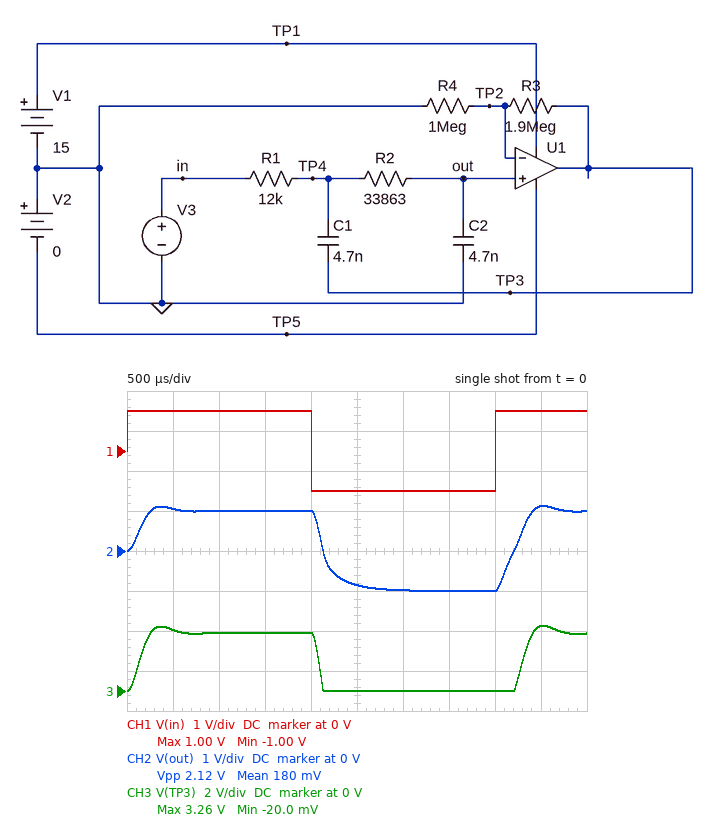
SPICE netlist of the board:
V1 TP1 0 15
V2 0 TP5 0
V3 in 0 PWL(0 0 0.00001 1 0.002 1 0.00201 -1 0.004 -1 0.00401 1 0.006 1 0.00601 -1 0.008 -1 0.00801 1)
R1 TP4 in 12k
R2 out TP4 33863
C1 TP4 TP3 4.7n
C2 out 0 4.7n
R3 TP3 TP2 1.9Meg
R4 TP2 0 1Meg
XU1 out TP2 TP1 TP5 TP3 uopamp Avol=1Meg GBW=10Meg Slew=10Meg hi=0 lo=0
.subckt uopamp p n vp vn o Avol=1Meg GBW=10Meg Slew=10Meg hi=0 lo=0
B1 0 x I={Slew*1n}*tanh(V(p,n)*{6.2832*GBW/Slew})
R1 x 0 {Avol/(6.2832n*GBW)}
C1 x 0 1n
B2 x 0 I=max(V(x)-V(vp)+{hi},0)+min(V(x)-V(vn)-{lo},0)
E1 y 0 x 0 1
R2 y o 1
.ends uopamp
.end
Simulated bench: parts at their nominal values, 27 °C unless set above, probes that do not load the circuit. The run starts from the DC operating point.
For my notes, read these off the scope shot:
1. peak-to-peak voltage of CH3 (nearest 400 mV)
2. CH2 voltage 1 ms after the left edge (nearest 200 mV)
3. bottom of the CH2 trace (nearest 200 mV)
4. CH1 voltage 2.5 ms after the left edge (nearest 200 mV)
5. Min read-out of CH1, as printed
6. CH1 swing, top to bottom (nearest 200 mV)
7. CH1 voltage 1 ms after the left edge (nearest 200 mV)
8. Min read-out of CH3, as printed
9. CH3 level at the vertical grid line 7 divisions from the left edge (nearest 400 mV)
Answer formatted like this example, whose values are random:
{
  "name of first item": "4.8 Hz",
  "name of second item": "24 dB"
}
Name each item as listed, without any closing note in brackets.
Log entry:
{
  "peak-to-peak voltage of CH3": "3.2 V",
  "CH2 voltage 1 ms after the left edge": "1.0 V",
  "bottom of the CH2 trace": "-1.0 V",
  "CH1 voltage 2.5 ms after the left edge": "-1.0 V",
  "Min read-out of CH1, as printed": "-1.00 V",
  "CH1 swing, top to bottom": "2.0 V",
  "CH1 voltage 1 ms after the left edge": "1.0 V",
  "Min read-out of CH3, as printed": "-20.0 mV",
  "CH3 level at the vertical grid line 7 divisions from the left edge": "0 V"
}
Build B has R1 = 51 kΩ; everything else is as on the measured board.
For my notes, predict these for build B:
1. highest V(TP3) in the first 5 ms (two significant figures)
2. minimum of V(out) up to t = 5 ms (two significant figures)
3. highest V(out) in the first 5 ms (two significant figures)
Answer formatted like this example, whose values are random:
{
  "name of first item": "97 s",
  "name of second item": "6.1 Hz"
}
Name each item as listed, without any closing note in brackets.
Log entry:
{
  "highest V(TP3) in the first 5 ms": "7.7 V",
  "minimum of V(out) up to t = 5 ms": "-1.2 V",
  "highest V(out) in the first 5 ms": "2.7 V"
}
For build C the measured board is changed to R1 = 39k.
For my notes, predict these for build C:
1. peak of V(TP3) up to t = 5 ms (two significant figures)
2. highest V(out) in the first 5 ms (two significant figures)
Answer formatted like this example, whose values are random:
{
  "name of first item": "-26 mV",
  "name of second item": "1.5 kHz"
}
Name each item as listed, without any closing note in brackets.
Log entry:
{
  "peak of V(TP3) up to t = 5 ms": "6.2 V",
  "highest V(out) in the first 5 ms": "2.1 V"
}
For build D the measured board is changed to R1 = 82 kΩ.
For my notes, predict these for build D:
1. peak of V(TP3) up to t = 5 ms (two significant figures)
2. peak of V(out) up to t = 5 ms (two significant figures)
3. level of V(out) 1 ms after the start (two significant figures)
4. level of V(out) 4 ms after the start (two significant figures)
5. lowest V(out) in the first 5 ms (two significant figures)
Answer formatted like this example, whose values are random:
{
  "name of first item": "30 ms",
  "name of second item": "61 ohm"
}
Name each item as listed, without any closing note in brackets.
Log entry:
{
  "peak of V(TP3) up to t = 5 ms": "13 V",
  "peak of V(out) up to t = 5 ms": "4.6 V",
  "level of V(out) 1 ms after the start": "3.8 V",
  "level of V(out) 4 ms after the start": "-910 mV",
  "lowest V(out) in the first 5 ms": "-1.4 V"
}
